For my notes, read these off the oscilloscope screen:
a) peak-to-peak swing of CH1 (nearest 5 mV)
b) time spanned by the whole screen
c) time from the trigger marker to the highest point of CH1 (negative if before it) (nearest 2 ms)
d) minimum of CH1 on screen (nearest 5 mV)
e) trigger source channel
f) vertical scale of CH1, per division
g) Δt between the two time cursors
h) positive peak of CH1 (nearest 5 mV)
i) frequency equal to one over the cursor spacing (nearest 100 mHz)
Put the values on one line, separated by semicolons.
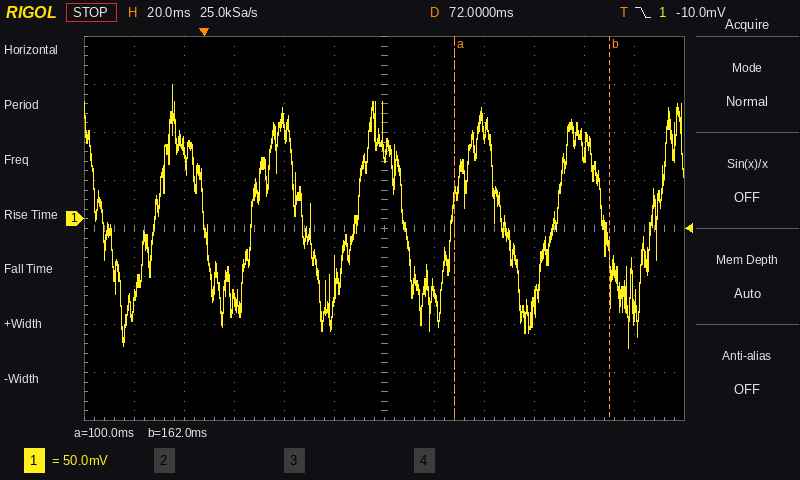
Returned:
275 mV; 240 ms; -12 ms; -135 mV; CH1; 50 mV; 62 ms; 140 mV; 16.1 Hz
